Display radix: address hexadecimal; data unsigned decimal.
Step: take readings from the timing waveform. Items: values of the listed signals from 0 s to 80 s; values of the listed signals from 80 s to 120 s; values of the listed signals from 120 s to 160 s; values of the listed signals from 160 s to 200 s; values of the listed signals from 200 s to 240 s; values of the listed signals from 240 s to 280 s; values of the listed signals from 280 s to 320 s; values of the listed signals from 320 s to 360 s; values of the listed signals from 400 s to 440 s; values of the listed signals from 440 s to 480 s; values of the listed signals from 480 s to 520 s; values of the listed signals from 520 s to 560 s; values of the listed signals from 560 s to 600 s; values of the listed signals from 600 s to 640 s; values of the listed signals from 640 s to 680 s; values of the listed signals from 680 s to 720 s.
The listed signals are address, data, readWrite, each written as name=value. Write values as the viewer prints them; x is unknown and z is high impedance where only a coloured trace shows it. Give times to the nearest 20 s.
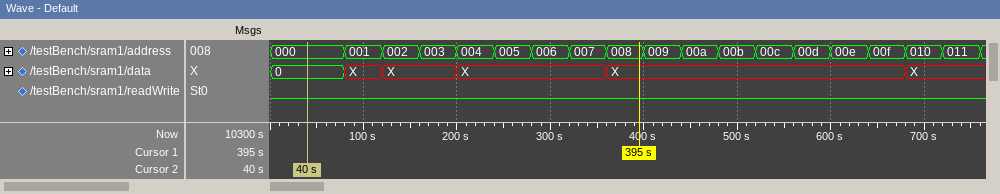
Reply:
address=000, data=0, readWrite=0
address=001, data=X, readWrite=0
address=002, data=X, readWrite=0
address=003, data=X, readWrite=0
address=004, data=X, readWrite=0
address=005, data=X, readWrite=0
address=006, data=X, readWrite=0
address=007, data=X, readWrite=0
address=009, data=X, readWrite=0
address=00a, data=X, readWrite=0
address=00b, data=X, readWrite=0
address=00c, data=X, readWrite=0
address=00d, data=X, readWrite=0
address=00e, data=X, readWrite=0
address=00f, data=X, readWrite=0
address=010, data=X, readWrite=0
